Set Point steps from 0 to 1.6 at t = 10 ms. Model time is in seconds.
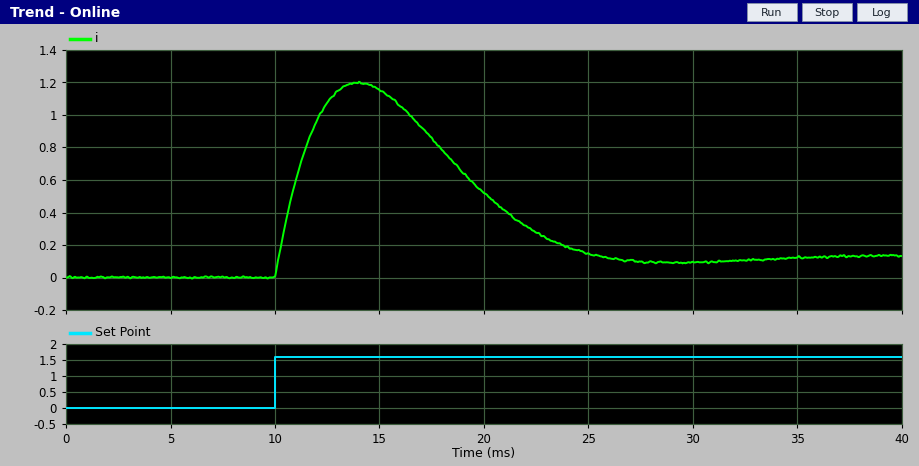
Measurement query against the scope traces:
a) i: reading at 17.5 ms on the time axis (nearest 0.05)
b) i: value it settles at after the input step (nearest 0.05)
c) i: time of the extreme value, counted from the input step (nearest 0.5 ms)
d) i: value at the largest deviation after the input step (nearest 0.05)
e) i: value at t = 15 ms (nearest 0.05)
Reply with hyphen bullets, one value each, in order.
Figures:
- 0.85
- 0.15
- 4.0 ms
- 1.20
- 1.15
